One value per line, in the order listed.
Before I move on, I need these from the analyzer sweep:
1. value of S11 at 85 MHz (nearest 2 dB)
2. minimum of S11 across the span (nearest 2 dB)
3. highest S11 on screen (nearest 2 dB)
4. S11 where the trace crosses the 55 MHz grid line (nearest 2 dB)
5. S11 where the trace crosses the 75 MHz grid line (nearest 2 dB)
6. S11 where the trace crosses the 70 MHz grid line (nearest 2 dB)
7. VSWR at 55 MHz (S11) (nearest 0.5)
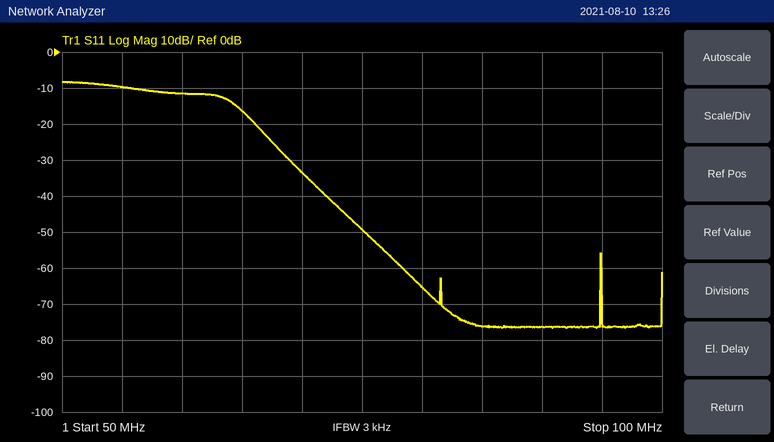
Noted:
-76 dB
-76 dB
-8 dB
-10 dB
-50 dB
-34 dB
2.0
